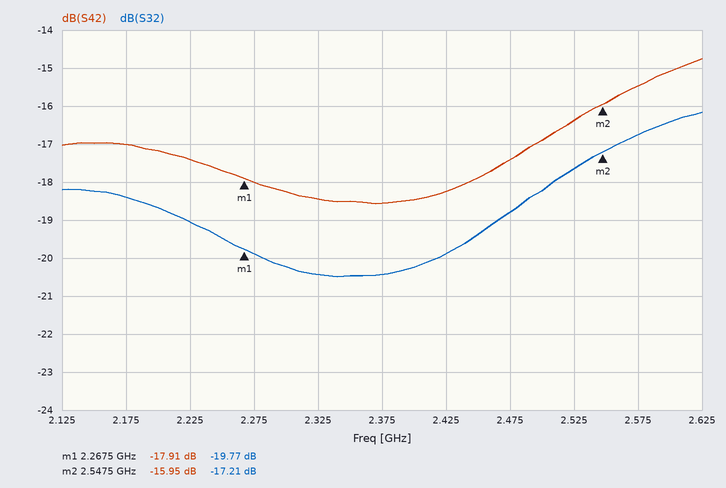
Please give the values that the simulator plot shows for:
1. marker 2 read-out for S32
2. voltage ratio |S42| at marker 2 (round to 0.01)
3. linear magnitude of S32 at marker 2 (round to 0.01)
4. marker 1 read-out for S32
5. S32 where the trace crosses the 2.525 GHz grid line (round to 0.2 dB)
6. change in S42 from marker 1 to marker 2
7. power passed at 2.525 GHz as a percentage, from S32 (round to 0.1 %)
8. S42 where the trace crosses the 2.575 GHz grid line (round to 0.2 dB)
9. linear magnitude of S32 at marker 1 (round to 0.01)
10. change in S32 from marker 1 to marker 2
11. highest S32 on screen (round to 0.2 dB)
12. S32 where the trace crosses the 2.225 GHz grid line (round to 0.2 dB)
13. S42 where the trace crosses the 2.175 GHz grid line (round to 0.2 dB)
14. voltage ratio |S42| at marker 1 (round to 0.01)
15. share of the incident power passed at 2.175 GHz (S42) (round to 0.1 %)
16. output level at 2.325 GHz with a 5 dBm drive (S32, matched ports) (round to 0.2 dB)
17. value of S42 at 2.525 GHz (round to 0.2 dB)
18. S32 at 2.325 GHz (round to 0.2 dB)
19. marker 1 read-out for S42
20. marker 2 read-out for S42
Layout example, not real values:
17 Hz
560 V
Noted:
-17.21 dB
0.16
0.14
-19.77 dB
-17.6 dB
1.96 dB
1.7 %
-15.4 dB
0.10
2.56 dB
-16.2 dB
-19.0 dB
-17.0 dB
0.13
2.0 %
-15.4 dBm
-16.4 dB
-20.4 dB
-17.91 dB
-15.95 dB
